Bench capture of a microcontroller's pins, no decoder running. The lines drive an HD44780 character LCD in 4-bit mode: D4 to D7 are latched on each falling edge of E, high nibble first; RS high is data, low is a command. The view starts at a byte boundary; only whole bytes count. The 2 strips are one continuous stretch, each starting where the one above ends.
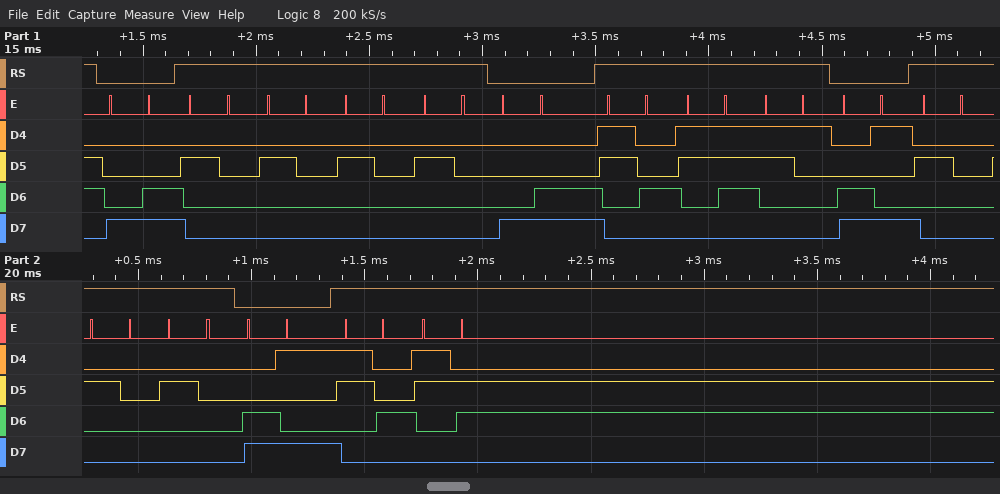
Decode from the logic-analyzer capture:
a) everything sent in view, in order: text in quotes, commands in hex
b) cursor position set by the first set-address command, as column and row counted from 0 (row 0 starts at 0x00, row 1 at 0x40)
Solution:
0x8C "    " 0x8C "471" 0xC9 "   " 0xC9 "46"
column 12, row 0
